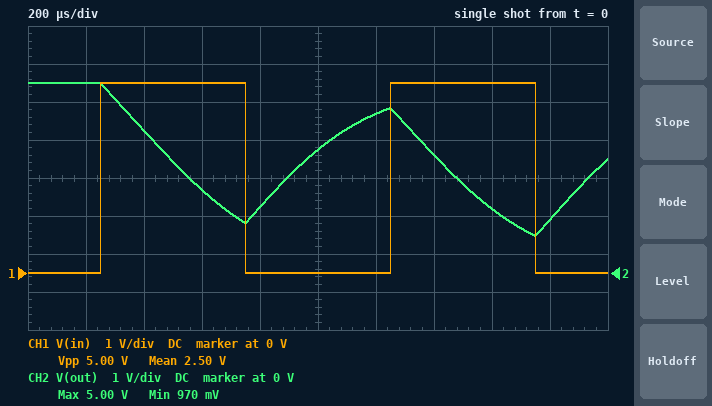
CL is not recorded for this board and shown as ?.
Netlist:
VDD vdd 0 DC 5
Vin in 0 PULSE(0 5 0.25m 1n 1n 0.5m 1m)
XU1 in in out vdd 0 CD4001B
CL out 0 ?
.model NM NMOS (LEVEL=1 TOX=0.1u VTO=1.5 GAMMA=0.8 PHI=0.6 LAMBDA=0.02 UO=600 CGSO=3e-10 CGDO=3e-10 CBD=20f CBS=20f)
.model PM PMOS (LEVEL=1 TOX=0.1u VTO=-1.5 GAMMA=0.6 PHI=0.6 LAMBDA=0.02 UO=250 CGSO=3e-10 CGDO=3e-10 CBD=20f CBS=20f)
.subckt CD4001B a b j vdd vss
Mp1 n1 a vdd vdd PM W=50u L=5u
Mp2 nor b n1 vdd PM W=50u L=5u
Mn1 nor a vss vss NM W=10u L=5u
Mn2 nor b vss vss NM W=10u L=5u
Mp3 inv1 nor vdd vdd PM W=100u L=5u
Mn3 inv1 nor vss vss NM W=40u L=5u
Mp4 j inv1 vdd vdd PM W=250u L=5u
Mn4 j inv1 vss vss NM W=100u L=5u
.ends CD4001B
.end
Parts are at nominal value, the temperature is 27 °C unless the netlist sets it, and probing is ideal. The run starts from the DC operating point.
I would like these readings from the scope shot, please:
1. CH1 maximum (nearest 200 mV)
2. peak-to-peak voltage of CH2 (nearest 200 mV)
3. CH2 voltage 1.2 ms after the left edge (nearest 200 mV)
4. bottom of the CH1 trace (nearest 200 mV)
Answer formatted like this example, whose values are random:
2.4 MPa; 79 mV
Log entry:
5.0 V; 4.0 V; 4.2 V; 0 V
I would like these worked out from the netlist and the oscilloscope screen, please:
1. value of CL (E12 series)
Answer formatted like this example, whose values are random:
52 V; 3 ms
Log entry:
330 nF
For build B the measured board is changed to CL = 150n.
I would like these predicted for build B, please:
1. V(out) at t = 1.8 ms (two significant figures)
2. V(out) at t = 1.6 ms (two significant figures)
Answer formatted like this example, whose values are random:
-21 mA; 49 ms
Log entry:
1.1 V; 430 mV
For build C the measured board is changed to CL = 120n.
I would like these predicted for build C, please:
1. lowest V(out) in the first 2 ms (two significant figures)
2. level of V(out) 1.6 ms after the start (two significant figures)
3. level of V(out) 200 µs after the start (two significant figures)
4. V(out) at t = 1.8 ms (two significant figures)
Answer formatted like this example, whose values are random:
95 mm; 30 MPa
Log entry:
33 mV; 200 mV; 5.0 V; 1.2 V
